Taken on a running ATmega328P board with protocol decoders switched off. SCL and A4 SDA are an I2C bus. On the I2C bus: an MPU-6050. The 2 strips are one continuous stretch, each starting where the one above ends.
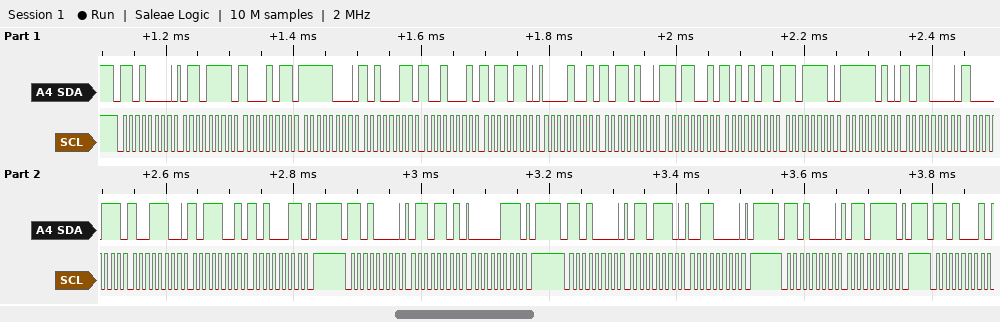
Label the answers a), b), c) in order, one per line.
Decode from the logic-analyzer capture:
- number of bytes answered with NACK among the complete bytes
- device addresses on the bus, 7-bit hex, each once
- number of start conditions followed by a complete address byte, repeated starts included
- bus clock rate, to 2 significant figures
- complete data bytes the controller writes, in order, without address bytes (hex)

a) 0
b) 0x68
c) 5
d) 100 kHz
e) 6F 8B F8 A3 91 B6 09 B4 D9 AB DE FA B0 87 9C B9 A3 6D 07 6E 30 6F
